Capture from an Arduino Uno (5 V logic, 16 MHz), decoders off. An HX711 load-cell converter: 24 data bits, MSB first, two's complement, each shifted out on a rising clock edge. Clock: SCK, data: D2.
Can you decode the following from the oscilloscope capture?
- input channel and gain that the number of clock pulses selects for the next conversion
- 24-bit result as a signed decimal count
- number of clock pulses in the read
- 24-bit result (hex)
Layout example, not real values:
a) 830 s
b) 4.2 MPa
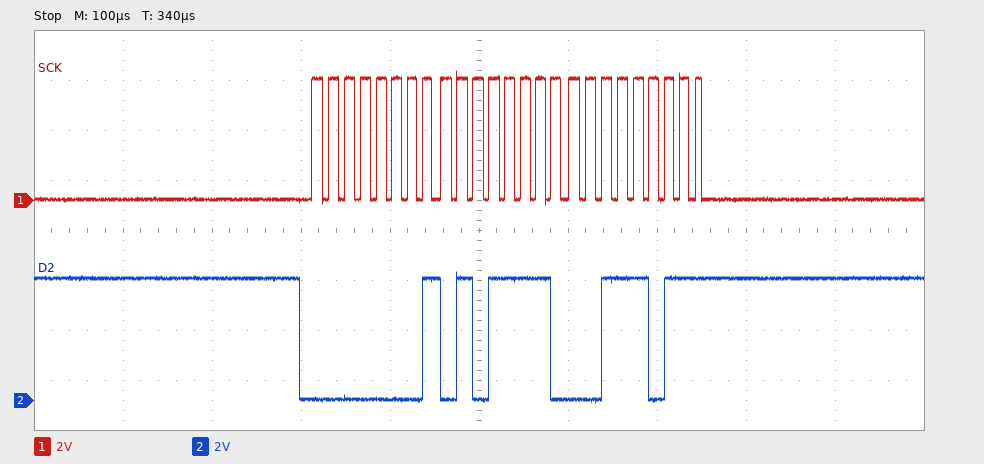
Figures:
a) channel A, gain 128
b) 89659
c) 25
d) 0x015E3B
